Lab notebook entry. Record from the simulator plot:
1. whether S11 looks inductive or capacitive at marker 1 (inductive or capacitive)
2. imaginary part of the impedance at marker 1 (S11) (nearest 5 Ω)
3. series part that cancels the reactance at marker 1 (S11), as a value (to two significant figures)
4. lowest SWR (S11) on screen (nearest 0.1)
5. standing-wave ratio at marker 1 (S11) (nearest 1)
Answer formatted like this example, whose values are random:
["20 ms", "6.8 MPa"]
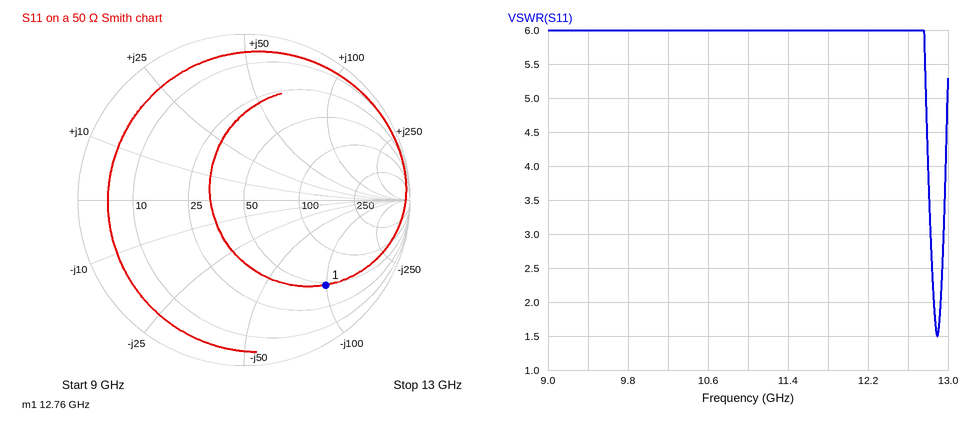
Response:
["capacitive", "-100 Ω", "1.2 nH", "1.5", "6"]
